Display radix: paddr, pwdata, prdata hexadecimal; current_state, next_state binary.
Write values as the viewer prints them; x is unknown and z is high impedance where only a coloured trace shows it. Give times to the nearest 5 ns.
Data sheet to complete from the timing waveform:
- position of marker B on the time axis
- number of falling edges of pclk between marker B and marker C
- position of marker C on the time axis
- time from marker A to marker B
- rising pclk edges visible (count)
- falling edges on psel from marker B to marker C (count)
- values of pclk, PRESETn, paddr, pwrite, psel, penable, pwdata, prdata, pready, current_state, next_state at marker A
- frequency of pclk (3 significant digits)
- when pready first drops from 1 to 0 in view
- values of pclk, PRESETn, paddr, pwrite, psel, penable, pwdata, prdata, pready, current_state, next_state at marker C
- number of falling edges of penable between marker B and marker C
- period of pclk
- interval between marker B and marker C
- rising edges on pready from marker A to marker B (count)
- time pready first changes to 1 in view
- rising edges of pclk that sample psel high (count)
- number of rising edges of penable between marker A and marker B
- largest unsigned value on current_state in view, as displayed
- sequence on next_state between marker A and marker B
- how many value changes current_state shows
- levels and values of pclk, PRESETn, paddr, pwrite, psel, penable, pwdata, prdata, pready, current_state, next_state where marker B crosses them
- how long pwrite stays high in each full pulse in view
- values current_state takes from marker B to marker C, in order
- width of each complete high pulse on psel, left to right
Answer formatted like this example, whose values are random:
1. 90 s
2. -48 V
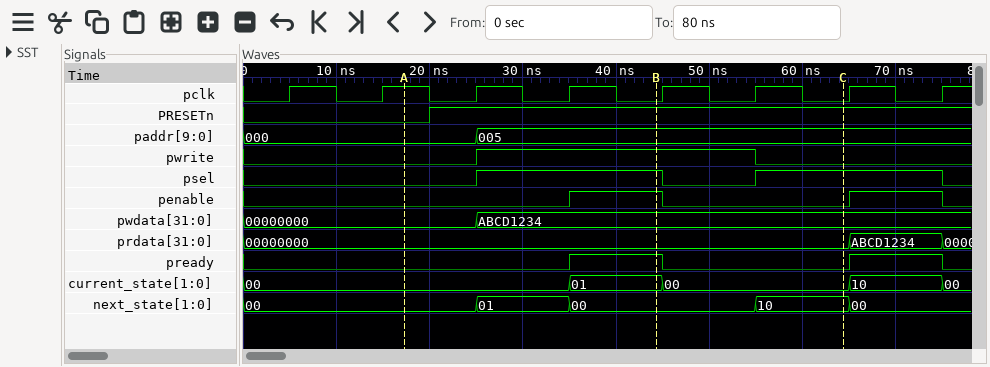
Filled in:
1. 45 ns
2. 2
3. 65 ns
4. 25 ns
5. 8
6. 1
7. pclk=1, PRESETn=0, paddr=000, pwrite=0, psel=0, penable=0, pwdata=00000000, prdata=00000000, pready=0, current_state=00, next_state=00
8. 100 MHz
9. 45 ns
10. pclk=0, PRESETn=1, paddr=005, pwrite=0, psel=1, penable=0, pwdata=ABCD1234, prdata=00000000, pready=0, current_state=00, next_state=10
11. 1
12. 10 ns
13. 20 ns
14. 1
15. 35 ns
16. 4
17. 1
18. 10
19. 00, 01, 00
20. 4
21. pclk=0, PRESETn=1, paddr=005, pwrite=1, psel=1, penable=1, pwdata=ABCD1234, prdata=00000000, pready=1, current_state=01, next_state=00
22. 30 ns
23. 01, 00
24. 20 ns, 20 ns
